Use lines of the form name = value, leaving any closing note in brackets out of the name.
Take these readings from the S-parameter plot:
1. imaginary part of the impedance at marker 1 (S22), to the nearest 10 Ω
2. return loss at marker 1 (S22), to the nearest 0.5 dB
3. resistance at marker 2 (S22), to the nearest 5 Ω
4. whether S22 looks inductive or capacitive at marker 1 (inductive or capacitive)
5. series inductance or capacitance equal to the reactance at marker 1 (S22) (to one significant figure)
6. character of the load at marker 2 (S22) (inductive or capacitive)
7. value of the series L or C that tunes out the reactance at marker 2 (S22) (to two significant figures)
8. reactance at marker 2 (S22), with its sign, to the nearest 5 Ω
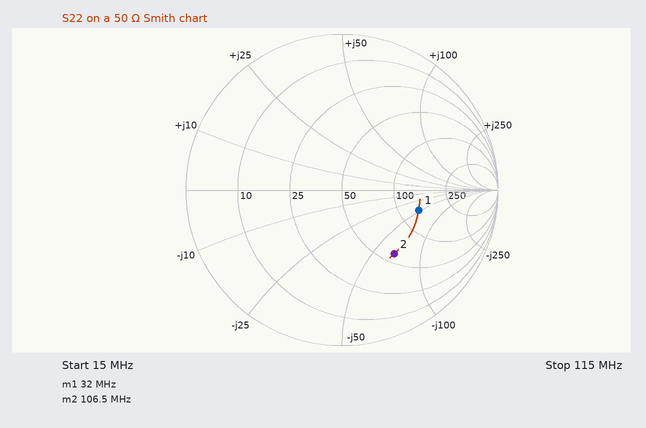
imaginary part of the impedance at marker 1 (S22), to the nearest 10 Ω = -50 Ω
return loss at marker 1 (S22), to the nearest 0.5 dB = 6.0 dB
resistance at marker 2 (S22), to the nearest 5 Ω = 60 Ω
whether S22 looks inductive or capacitive at marker 1 = capacitive
series inductance or capacitance equal to the reactance at marker 1 (S22) = 100 pF
character of the load at marker 2 (S22) = capacitive
value of the series L or C that tunes out the reactance at marker 2 (S22) = 100 nH
reactance at marker 2 (S22), with its sign, to the nearest 5 Ω = -65 Ω
